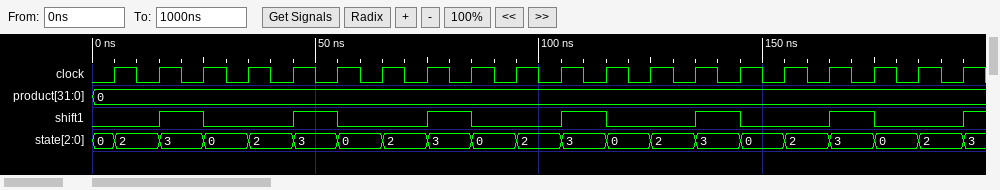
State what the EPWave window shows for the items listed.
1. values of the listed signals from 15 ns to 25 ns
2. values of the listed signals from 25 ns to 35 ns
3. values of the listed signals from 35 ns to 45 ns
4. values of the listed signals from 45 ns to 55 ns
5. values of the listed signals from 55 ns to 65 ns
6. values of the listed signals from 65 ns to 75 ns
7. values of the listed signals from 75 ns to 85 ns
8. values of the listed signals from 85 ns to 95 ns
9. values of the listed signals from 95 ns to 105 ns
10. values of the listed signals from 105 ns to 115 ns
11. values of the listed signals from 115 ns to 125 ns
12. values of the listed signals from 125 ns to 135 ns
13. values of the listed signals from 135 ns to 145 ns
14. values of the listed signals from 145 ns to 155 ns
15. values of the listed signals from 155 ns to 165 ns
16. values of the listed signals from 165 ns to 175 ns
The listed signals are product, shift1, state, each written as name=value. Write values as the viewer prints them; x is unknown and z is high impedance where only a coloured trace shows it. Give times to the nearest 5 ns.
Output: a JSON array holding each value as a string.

["product=0, shift1=1, state=3", "product=0, shift1=0, state=0", "product=0, shift1=0, state=2", "product=0, shift1=1, state=3", "product=0, shift1=0, state=0", "product=0, shift1=0, state=2", "product=0, shift1=1, state=3", "product=0, shift1=0, state=0", "product=0, shift1=0, state=2", "product=0, shift1=1, state=3", "product=0, shift1=0, state=0", "product=0, shift1=0, state=2", "product=0, shift1=1, state=3", "product=0, shift1=0, state=0", "product=0, shift1=0, state=2", "product=0, shift1=1, state=3"]
